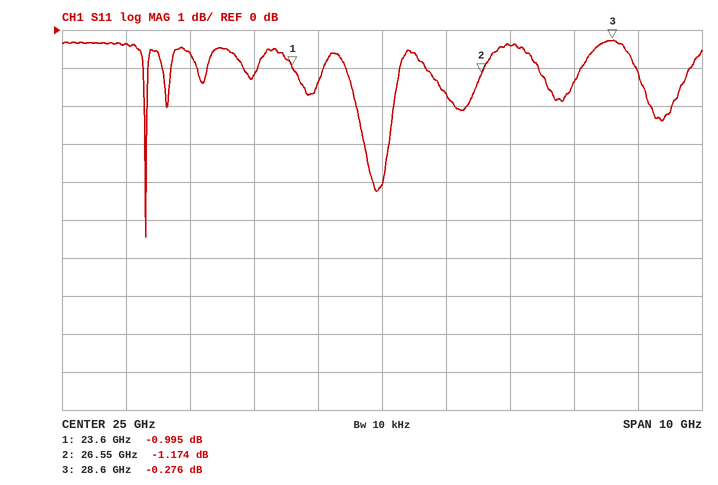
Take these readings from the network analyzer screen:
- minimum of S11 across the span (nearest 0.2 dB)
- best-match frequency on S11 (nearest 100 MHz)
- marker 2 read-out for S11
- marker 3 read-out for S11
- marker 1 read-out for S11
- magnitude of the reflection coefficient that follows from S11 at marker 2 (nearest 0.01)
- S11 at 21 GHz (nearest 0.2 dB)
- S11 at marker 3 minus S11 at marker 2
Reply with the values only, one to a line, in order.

-5.4 dB
21.3 GHz
-1.174 dB
-0.276 dB
-0.995 dB
0.87
-0.4 dB
0.898 dB
